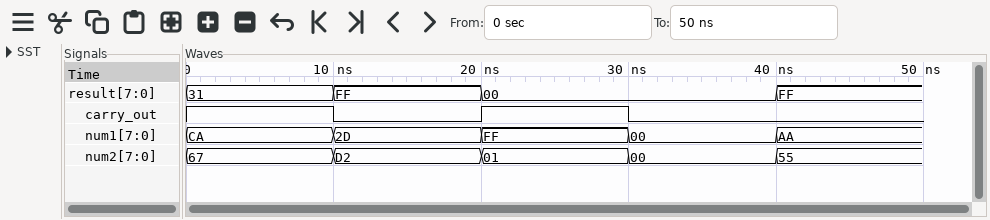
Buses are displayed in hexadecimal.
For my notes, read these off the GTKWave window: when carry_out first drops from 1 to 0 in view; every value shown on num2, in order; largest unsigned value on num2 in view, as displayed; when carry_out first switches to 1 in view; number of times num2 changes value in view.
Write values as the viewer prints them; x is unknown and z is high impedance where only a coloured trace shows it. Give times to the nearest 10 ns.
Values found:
10 ns
67, D2, 01, 00, 55
D2
20 ns
4
